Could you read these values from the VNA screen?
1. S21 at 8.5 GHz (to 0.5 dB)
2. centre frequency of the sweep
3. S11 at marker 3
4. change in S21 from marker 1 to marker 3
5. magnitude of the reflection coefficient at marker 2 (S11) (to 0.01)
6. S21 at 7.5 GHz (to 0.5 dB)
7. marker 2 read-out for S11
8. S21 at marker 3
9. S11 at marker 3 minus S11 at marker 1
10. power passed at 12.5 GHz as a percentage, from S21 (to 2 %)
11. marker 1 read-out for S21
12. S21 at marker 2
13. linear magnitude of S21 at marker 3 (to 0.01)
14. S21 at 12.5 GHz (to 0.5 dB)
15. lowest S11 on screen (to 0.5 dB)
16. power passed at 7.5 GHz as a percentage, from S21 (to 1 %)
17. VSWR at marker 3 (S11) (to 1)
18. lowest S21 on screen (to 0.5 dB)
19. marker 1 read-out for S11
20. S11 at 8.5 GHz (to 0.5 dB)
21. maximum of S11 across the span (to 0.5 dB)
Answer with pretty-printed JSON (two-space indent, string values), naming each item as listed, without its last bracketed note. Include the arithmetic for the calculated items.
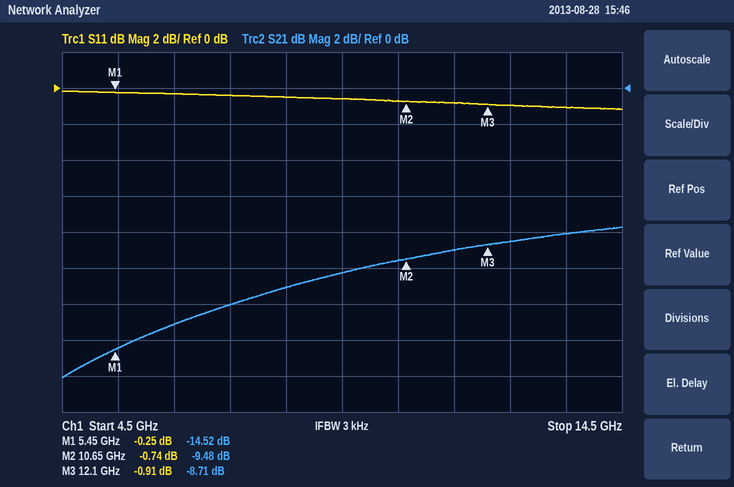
{
  "S21 at 8.5 GHz": "-11.0 dB",
  "centre frequency of the sweep": "9.5 GHz",
  "S11 at marker 3": "-0.91 dB",
  "change in S21 from marker 1 to marker 3": "-8.71 − (-14.52) = 5.81 dB",
  "magnitude of the reflection coefficient at marker 2 (S11)": "10^(-0.74/20) ≈ 0.92",
  "S21 at 7.5 GHz": "-12.0 dB",
  "marker 2 read-out for S11": "-0.74 dB",
  "S21 at marker 3": "-8.71 dB",
  "S11 at marker 3 minus S11 at marker 1": "-0.91 − (-0.25) = -0.66 dB",
  "power passed at 12.5 GHz as a percentage, from S21": "10^(-8.5/10) ≈ 14 %",
  "marker 1 read-out for S21": "-14.52 dB",
  "S21 at marker 2": "-9.48 dB",
  "linear magnitude of S21 at marker 3": "10^(-8.71/20) ≈ 0.37",
  "S21 at 12.5 GHz": "-8.5 dB",
  "lowest S11 on screen": "-1.0 dB",
  "power passed at 7.5 GHz as a percentage, from S21": "10^(-12/10) ≈ 6 %",
  "VSWR at marker 3 (S11)": "(1 + 0.9005)/(1 − 0.9005) ≈ 19",
  "lowest S21 on screen": "-16.0 dB",
  "marker 1 read-out for S11": "-0.25 dB",
  "S11 at 8.5 GHz": "-0.5 dB",
  "maximum of S11 across the span": "0.0 dB"
}
